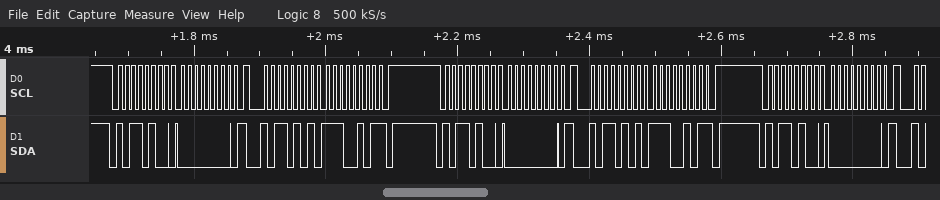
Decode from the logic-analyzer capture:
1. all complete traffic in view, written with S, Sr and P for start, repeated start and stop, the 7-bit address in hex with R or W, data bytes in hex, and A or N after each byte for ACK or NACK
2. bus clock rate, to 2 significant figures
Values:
S 5AW A 00 A Sr 5AR A E5 N P S 5AW A 00 A Sr 5AR A E5 N P S 5AW A 00 A
100 kHz
